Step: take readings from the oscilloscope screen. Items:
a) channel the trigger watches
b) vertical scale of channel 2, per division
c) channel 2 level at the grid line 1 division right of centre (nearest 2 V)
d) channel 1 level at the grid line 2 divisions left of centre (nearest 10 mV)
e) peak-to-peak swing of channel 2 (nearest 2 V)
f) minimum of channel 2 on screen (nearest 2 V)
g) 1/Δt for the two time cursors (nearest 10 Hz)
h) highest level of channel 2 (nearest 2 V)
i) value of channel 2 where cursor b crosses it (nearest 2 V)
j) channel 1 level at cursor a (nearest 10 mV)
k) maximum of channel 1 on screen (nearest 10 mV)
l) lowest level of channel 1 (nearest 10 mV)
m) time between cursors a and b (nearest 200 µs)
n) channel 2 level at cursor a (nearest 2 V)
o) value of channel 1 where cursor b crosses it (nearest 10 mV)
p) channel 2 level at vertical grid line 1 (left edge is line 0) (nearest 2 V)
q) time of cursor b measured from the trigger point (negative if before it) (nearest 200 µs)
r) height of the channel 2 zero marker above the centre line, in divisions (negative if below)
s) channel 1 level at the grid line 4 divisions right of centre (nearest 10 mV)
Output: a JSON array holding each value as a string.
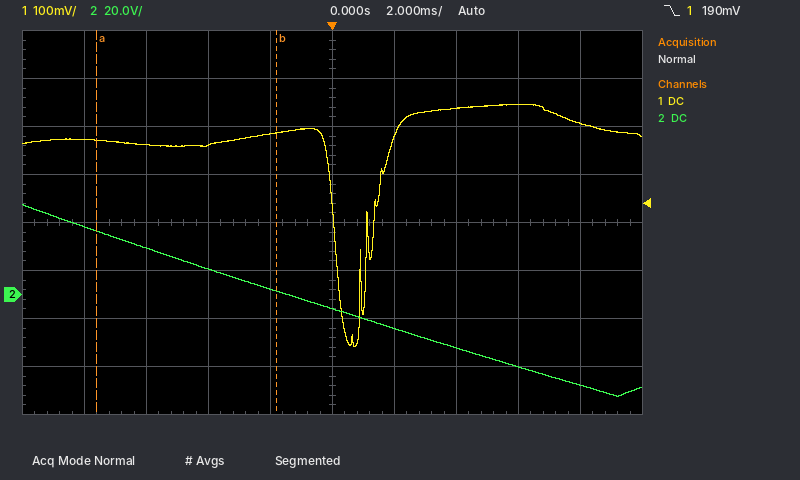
["channel 1", "20 V", "-14 V", "310 mV", "80 V", "-42 V", "170 Hz", "38 V", "2 V", "320 mV", "400 mV", "-110 mV", "5.8 ms", "26 V", "340 mV", "28 V", "-1.8 ms", "-1.5 div", "360 mV"]
